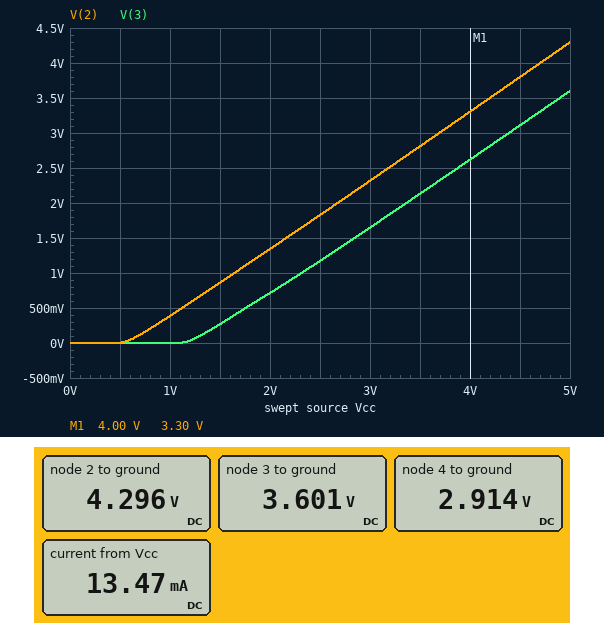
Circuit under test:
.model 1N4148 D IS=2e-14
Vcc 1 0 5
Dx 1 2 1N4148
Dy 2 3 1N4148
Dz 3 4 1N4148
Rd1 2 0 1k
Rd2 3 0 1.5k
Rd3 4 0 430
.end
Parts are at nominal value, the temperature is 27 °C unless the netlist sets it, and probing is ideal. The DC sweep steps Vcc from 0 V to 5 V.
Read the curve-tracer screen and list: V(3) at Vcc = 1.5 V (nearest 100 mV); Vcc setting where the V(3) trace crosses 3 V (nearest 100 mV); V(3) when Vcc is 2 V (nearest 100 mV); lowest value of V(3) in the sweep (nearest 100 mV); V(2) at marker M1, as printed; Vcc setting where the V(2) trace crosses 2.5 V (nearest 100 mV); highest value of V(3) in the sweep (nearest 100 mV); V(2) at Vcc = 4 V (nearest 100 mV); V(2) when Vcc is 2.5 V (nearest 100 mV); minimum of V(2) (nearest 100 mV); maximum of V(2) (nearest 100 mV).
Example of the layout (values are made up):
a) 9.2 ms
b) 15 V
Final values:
a) 300 mV
b) 4.4 V
c) 700 mV
d) 0 V
e) 3.30 V
f) 3.2 V
g) 3.6 V
h) 3.3 V
i) 1.8 V
j) 0 V
k) 4.3 V
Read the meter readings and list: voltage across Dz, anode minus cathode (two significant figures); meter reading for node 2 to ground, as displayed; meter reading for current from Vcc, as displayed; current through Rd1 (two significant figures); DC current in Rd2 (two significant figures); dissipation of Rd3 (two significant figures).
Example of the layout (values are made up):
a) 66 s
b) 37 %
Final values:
a) 690 mV
b) 4.296 V
c) 13.47 mA
d) 4.3 mA
e) 2.4 mA
f) 20 mW
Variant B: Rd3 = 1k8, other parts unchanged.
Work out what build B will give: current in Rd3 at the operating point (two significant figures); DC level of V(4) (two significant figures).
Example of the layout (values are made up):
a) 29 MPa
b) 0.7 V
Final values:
a) 1.7 mA
b) 3.0 V
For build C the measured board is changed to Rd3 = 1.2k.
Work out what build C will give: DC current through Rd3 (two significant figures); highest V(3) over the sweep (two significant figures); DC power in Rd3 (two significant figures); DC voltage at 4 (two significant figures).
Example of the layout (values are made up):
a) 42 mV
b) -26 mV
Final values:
a) 2.5 mA
b) 3.6 V
c) 7.3 mW
d) 3.0 V
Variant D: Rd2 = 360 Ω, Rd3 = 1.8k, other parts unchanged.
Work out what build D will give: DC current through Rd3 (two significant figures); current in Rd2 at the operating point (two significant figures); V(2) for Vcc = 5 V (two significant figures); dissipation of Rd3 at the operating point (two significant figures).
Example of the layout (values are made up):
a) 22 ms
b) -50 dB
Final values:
a) 1.6 mA
b) 10 mA
c) 4.3 V
d) 4.8 mW
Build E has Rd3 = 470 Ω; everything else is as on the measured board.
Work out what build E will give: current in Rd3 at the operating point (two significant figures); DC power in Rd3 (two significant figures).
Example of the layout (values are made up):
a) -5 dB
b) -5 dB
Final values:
a) 6.2 mA
b) 18 mW
